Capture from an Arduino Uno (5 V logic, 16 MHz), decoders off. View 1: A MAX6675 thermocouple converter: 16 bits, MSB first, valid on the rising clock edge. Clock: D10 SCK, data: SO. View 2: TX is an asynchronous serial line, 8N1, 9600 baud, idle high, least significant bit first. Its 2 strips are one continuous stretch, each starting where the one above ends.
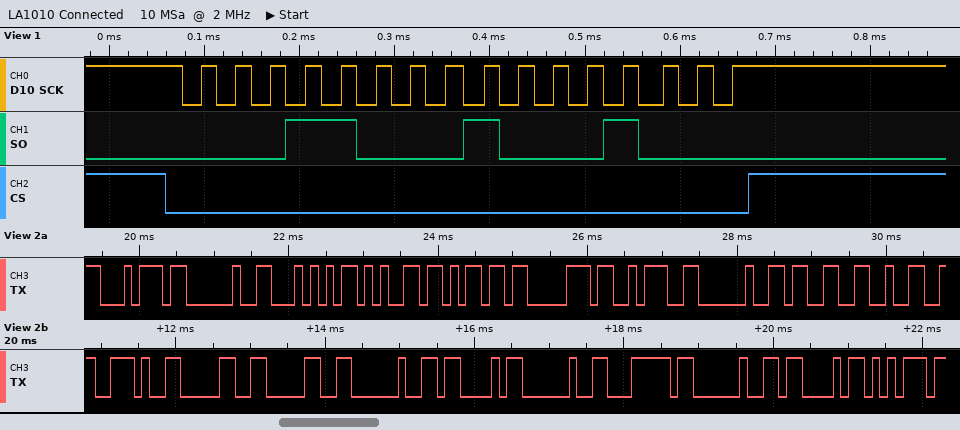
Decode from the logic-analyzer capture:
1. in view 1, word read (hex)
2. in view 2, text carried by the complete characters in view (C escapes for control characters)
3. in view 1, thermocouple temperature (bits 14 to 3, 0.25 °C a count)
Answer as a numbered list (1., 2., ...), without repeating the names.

1. 0x1888
2. "t Temp: 32.00 C | Cu"
3. 196.25 °C
